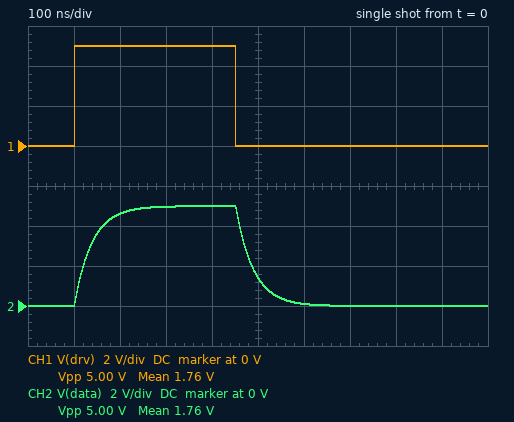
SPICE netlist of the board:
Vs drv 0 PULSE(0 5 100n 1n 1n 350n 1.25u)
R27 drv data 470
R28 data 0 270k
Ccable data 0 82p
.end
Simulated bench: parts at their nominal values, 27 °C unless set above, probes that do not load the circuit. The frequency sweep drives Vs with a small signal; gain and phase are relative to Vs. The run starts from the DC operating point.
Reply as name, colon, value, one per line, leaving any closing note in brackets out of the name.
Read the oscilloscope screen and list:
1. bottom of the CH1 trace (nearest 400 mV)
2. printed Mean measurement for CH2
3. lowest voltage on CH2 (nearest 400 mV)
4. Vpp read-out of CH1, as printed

bottom of the CH1 trace: 0 V
printed Mean measurement for CH2: 1.76 V
lowest voltage on CH2: 0 V
Vpp read-out of CH1, as printed: 5.00 V
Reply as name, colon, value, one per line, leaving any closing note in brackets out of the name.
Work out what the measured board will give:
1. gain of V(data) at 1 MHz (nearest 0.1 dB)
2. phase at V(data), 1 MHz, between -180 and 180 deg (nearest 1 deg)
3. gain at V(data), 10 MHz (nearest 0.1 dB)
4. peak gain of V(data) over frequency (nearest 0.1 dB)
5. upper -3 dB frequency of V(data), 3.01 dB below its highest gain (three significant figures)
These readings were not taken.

gain of V(data) at 1 MHz: -0.3 dB
phase at V(data), 1 MHz, between -180 and 180 deg: -14 deg
gain at V(data), 10 MHz: -8.4 dB
peak gain of V(data) over frequency: 0 dB
upper -3 dB frequency of V(data), 3.01 dB below its highest gain: 4.14 MHz
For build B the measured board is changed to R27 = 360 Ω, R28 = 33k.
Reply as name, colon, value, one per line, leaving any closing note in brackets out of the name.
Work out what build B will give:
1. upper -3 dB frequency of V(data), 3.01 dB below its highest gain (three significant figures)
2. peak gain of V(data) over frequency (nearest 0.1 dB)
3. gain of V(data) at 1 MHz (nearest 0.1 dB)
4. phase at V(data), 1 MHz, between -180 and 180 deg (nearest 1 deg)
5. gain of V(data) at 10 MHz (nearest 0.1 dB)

upper -3 dB frequency of V(data), 3.01 dB below its highest gain: 5.45 MHz
peak gain of V(data) over frequency: -0.1 dB
gain of V(data) at 1 MHz: -0.2 dB
phase at V(data), 1 MHz, between -180 and 180 deg: -10 deg
gain of V(data) at 10 MHz: -6.5 dB
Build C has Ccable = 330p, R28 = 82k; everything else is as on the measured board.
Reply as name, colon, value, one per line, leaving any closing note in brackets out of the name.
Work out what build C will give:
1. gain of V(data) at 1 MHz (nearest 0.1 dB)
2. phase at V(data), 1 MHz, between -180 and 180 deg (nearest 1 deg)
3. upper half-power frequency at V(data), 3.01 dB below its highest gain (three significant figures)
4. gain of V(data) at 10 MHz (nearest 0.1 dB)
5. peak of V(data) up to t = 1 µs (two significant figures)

gain of V(data) at 1 MHz: -2.9 dB
phase at V(data), 1 MHz, between -180 and 180 deg: -44 deg
upper half-power frequency at V(data), 3.01 dB below its highest gain: 1.03 MHz
gain of V(data) at 10 MHz: -19.8 dB
peak of V(data) up to t = 1 µs: 4.5 V
